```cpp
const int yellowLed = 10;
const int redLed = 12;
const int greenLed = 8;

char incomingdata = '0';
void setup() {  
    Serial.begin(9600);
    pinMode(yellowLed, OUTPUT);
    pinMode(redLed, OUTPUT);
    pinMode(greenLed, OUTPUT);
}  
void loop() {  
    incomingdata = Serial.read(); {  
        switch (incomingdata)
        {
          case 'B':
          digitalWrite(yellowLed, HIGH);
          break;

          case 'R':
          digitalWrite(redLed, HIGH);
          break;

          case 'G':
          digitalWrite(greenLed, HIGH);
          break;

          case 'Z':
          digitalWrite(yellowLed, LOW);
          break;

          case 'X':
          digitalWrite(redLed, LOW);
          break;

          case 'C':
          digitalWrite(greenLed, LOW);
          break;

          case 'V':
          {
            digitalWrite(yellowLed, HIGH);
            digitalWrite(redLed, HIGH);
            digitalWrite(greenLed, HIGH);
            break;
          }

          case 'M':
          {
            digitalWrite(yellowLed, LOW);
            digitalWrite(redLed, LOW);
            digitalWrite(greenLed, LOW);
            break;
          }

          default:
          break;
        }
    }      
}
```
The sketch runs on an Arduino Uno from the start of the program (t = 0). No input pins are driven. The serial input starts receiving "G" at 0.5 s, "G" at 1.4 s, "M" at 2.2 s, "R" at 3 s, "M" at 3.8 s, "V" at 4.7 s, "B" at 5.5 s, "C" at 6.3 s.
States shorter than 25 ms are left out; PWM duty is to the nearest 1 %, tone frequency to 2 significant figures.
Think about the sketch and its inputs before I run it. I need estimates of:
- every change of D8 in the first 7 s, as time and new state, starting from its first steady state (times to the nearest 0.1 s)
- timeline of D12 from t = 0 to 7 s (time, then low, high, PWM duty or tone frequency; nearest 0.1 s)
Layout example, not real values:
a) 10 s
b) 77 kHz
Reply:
a) 0 s low; 0.5 s high; 2.2 s low; 4.7 s high; 6.3 s low
b) 0 s low; 3 s high; 3.8 s low; 4.7 s high
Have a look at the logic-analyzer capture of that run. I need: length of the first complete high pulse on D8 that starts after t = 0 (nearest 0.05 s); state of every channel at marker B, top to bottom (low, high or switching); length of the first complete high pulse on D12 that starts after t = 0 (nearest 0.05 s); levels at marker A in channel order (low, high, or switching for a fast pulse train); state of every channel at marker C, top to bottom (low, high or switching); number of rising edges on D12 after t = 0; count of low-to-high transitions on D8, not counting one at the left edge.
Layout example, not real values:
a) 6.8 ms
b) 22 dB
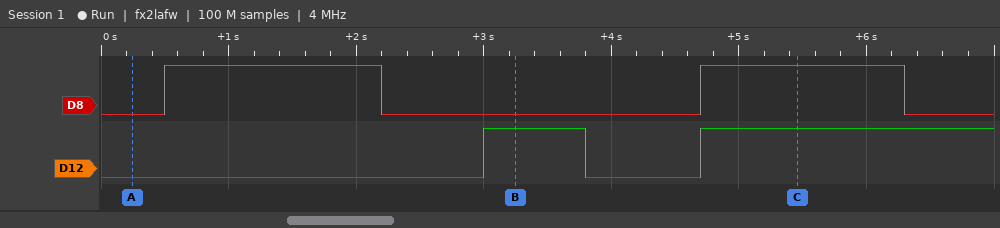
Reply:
a) 1.70 s
b) D8 low, D12 high
c) 0.80 s
d) D8 low, D12 low
e) D8 high, D12 high
f) 2
g) 2
